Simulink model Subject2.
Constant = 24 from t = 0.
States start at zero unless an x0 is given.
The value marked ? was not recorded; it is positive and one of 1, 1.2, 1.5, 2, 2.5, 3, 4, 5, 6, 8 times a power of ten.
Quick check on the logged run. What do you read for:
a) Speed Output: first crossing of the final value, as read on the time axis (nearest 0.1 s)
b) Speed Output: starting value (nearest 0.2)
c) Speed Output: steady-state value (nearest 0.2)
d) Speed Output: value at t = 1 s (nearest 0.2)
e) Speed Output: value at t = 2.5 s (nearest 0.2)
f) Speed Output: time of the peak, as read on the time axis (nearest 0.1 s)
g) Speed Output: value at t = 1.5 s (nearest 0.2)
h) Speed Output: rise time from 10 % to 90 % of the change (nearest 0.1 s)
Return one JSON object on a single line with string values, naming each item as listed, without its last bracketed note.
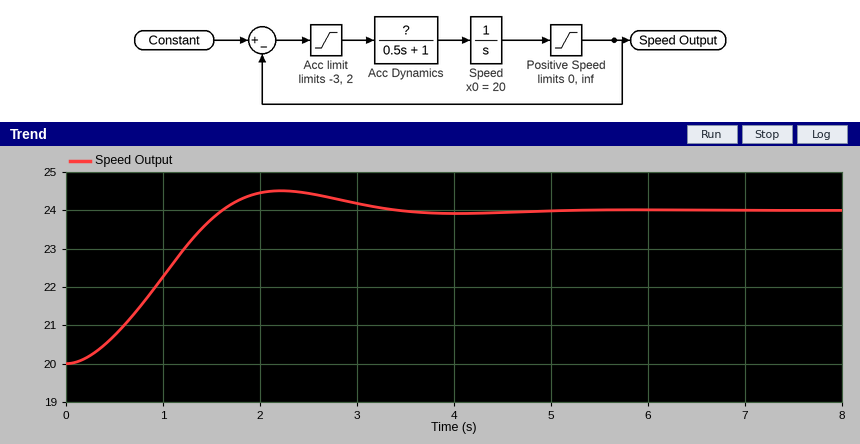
{"Speed Output: first crossing of the final value, as read on the time axis": "1.6 s", "Speed Output: starting value": "20.0", "Speed Output: steady-state value": "24.0", "Speed Output: value at t = 1 s": "22.2", "Speed Output: value at t = 2.5 s": "24.4", "Speed Output: time of the peak, as read on the time axis": "2.2 s", "Speed Output: value at t = 1.5 s": "23.8", "Speed Output: rise time from 10 % to 90 % of the change": "1.1 s"}
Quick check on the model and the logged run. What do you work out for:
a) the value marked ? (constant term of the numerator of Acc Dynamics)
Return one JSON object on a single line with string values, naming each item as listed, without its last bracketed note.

{"the value marked ?": "2"}
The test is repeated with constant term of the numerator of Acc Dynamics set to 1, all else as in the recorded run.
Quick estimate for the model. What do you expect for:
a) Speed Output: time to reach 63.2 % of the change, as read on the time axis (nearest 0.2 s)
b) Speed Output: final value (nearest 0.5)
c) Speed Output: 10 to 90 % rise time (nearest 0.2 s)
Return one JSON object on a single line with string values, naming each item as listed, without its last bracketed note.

{"Speed Output: time to reach 63.2 % of the change, as read on the time axis": "1.8 s", "Speed Output: final value": "24.0", "Speed Output: 10 to 90 % rise time": "2.0 s"}
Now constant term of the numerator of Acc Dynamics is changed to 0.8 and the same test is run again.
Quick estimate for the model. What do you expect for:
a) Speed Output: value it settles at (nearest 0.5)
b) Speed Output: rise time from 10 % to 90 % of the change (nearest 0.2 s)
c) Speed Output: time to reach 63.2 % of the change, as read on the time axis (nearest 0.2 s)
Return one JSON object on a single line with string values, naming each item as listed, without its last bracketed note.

{"Speed Output: value it settles at": "24.0", "Speed Output: rise time from 10 % to 90 % of the change": "2.4 s", "Speed Output: time to reach 63.2 % of the change, as read on the time axis": "2.0 s"}
